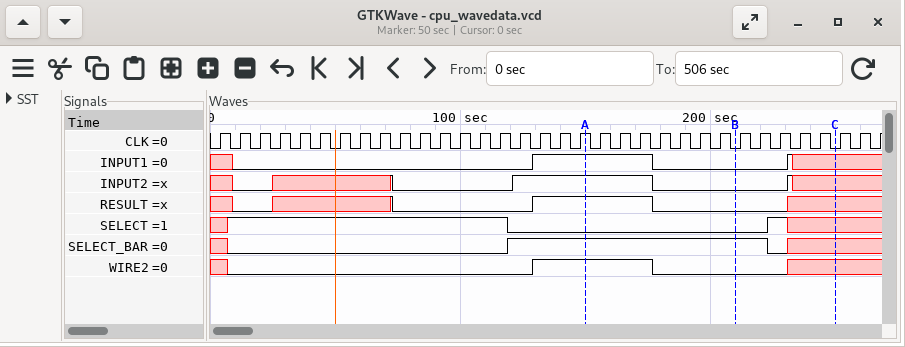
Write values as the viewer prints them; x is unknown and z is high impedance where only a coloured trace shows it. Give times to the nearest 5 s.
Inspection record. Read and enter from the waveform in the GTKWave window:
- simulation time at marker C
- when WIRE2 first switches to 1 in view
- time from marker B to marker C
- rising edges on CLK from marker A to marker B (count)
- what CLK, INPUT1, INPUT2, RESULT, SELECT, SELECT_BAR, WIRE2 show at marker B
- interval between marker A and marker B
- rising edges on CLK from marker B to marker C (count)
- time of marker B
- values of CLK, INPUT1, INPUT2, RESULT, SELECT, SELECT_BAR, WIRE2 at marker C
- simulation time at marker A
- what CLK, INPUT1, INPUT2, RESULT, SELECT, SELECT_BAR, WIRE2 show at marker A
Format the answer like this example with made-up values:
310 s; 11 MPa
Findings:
250 s; 130 s; 40 s; 7; CLK=0, INPUT1=0, INPUT2=0, RESULT=0, SELECT=0, SELECT_BAR=1, WIRE2=0; 60 s; 5; 210 s; CLK=0, INPUT1=x, INPUT2=x, RESULT=x, SELECT=x, SELECT_BAR=x, WIRE2=x; 150 s; CLK=1, INPUT1=1, INPUT2=1, RESULT=1, SELECT=0, SELECT_BAR=1, WIRE2=1
